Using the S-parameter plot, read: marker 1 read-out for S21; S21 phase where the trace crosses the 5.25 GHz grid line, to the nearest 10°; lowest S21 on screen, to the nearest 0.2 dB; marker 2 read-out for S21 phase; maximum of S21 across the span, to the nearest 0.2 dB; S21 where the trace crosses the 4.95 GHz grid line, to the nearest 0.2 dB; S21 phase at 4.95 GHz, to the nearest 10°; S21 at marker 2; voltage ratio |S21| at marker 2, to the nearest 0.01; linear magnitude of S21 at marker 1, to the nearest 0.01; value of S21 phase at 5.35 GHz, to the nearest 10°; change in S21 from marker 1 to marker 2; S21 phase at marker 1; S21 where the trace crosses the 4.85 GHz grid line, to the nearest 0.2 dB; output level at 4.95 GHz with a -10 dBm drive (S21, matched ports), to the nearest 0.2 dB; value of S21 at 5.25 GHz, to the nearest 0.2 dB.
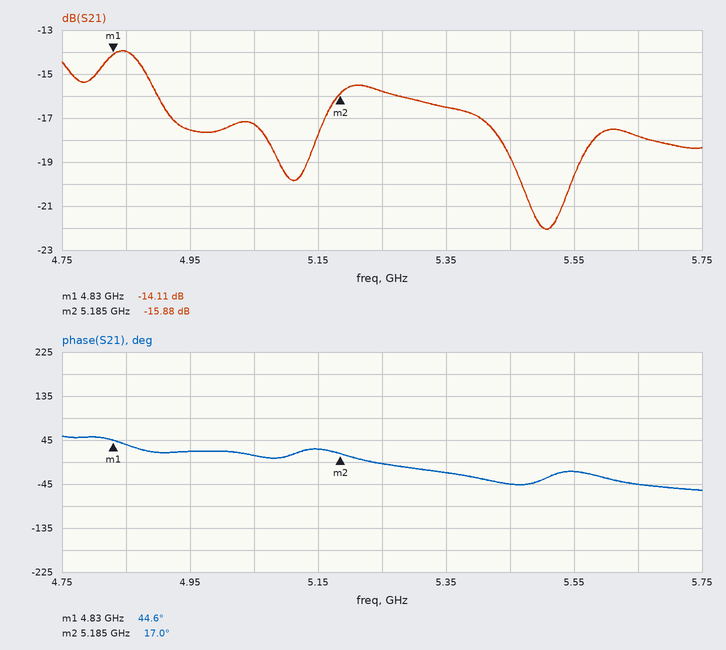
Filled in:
-14.11 dB
0°
-22.0 dB
17.0°
-14.0 dB
-17.6 dB
20°
-15.88 dB
0.16
0.20
-20°
-1.77 dB
44.6°
-14.0 dB
-27.6 dBm
-15.8 dB
